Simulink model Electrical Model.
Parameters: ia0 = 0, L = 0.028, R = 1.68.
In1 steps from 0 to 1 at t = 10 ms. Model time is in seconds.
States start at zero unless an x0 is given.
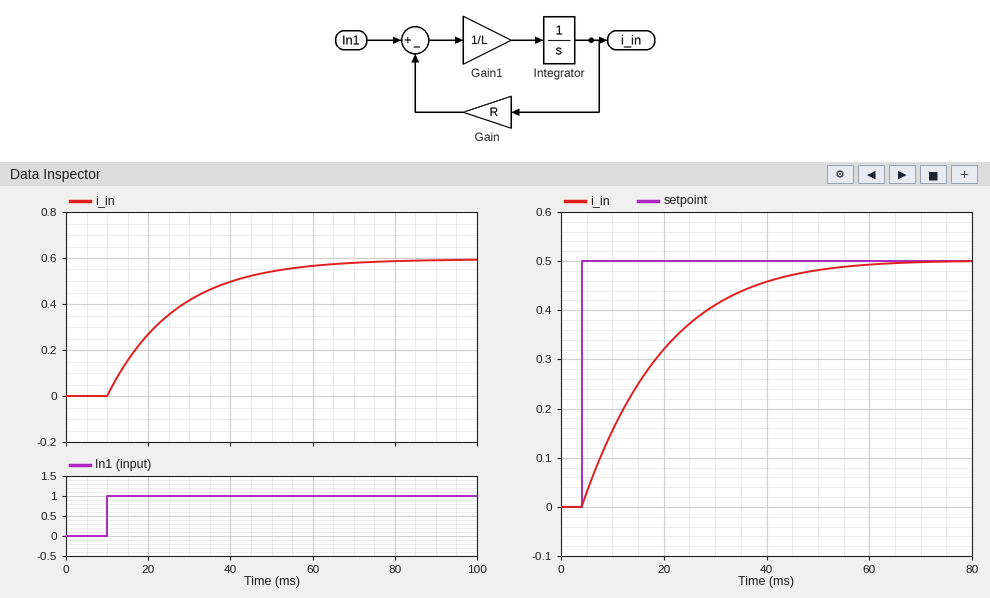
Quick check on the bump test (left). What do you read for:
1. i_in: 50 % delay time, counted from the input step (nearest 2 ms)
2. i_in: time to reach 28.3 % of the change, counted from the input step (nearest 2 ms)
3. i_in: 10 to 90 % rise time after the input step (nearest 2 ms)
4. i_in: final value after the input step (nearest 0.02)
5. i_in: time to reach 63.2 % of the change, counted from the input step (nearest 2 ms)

12 ms
6 ms
36 ms
0.60
16 ms
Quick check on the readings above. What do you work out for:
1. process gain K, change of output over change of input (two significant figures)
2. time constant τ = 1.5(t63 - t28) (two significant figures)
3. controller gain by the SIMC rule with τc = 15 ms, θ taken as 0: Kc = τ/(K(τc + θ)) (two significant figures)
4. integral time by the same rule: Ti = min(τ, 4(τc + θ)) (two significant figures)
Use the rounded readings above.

0.60
15 ms
1.7
15 ms
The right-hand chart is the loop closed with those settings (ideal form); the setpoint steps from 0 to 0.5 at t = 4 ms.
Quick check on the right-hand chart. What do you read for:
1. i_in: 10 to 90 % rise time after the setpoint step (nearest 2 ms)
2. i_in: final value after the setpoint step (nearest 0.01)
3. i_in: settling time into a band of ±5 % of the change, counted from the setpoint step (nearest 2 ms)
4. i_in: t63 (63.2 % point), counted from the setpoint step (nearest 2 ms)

32 ms
0.50
42 ms
16 ms
